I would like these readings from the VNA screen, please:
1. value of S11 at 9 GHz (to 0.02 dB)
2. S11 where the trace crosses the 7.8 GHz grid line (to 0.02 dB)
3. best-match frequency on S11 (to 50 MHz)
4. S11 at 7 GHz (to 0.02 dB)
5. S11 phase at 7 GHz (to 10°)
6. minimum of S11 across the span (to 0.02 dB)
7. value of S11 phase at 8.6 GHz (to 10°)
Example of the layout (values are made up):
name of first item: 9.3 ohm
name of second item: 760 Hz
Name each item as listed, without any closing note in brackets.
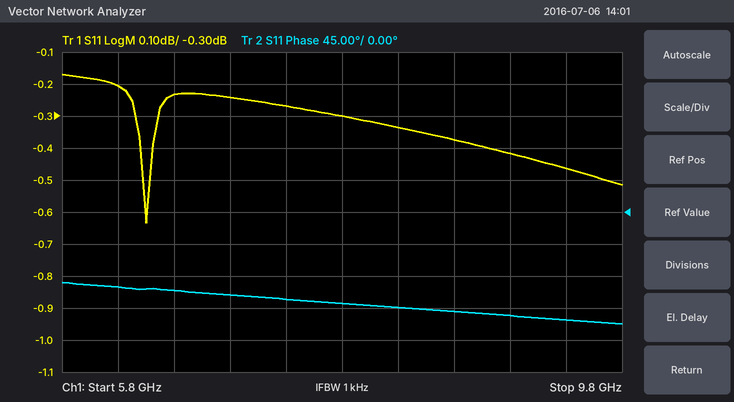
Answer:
value of S11 at 9 GHz: -0.42 dB
S11 where the trace crosses the 7.8 GHz grid line: -0.30 dB
best-match frequency on S11: 6.40 GHz
S11 at 7 GHz: -0.24 dB
S11 phase at 7 GHz: -120°
minimum of S11 across the span: -0.64 dB
value of S11 phase at 8.6 GHz: -140°
